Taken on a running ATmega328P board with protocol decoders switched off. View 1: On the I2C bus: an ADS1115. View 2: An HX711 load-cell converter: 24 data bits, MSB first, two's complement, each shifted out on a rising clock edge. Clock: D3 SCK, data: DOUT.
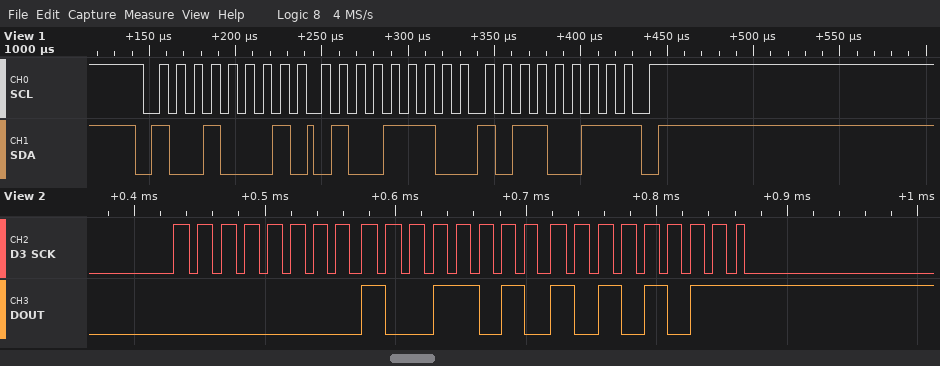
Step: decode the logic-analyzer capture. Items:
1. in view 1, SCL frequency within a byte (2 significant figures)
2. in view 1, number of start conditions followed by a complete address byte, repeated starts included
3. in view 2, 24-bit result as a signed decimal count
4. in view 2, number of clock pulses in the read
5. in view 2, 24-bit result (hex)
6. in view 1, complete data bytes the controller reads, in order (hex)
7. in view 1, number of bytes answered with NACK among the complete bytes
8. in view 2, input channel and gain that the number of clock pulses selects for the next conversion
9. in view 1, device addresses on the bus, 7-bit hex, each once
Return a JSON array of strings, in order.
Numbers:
["100 kHz", "1", "39595", "25", "0x009AAB", "4E B3", "1", "channel A, gain 128", "0x48"]
